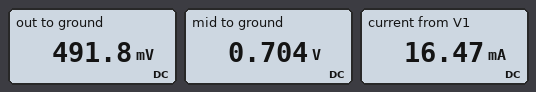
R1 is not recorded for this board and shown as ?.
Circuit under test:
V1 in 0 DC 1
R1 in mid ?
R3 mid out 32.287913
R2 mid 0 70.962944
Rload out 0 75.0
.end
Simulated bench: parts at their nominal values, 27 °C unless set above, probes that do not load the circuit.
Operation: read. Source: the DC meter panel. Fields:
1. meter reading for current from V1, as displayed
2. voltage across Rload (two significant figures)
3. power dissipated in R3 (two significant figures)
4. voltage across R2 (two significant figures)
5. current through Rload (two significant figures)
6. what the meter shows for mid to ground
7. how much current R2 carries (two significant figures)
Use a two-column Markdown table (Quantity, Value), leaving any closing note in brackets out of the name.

| Quantity | Value |
|---|---|
| meter reading for current from V1, as displayed | 16.47 mA |
| voltage across Rload | 490 mV |
| power dissipated in R3 | 1.4 mW |
| voltage across R2 | 700 mV |
| current through Rload | 6.6 mA |
| what the meter shows for mid to ground | 0.704 V |
| how much current R2 carries | 9.9 mA |
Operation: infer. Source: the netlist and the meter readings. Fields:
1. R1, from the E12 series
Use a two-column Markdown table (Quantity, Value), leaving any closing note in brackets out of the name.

| Quantity | Value |
|---|---|
| R1, from the E12 series | 18 Ω |
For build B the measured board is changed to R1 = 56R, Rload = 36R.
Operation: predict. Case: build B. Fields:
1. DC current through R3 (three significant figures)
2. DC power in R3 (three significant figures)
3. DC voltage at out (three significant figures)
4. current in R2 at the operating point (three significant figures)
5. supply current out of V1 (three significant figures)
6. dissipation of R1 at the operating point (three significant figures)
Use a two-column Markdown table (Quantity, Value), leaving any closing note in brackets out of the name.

| Quantity | Value |
|---|---|
| DC current through R3 | 5.61 mA |
| DC power in R3 | 1.02 mW |
| DC voltage at out | 202 mV |
| current in R2 at the operating point | 5.40 mA |
| supply current out of V1 | 11.0 mA |
| dissipation of R1 at the operating point | 6.79 mW |
